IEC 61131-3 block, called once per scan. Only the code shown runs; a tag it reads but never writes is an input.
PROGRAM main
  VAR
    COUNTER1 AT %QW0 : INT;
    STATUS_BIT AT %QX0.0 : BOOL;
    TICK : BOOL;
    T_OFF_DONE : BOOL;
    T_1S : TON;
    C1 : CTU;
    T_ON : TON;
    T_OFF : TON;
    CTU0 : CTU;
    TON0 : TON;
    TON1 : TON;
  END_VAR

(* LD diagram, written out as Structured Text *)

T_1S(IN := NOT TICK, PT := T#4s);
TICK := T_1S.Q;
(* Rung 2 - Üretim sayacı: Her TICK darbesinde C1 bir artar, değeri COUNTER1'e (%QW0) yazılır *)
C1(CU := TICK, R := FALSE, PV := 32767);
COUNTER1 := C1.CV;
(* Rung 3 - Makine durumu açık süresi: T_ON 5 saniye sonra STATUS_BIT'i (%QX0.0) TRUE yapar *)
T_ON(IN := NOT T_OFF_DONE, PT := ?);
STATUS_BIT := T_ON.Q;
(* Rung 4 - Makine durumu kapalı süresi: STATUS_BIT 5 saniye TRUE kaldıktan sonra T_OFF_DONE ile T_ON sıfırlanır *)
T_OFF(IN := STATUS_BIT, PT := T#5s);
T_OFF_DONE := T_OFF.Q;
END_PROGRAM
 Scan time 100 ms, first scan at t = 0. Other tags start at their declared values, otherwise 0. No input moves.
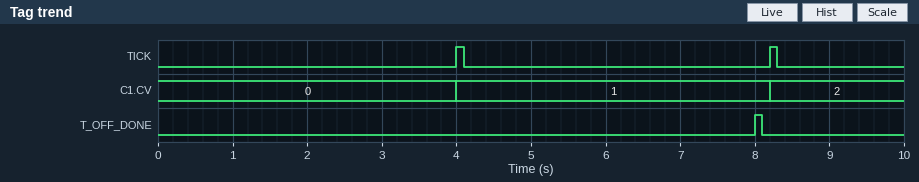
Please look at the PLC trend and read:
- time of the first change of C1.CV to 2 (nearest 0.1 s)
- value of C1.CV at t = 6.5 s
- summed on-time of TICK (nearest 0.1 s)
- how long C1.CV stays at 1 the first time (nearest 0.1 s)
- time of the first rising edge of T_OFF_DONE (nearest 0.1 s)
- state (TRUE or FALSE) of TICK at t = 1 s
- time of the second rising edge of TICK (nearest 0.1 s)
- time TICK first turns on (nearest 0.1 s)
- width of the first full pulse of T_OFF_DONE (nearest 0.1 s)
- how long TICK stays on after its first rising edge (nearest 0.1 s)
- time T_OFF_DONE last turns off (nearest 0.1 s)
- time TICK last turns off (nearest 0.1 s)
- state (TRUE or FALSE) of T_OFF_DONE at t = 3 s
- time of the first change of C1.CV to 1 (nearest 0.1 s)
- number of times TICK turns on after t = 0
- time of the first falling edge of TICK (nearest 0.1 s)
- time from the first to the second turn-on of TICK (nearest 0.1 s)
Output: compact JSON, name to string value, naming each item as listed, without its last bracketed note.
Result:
{"time of the first change of C1.CV to 2": "8.2 s", "value of C1.CV at t = 6.5 s": "1", "summed on-time of TICK": "0.2 s", "how long C1.CV stays at 1 the first time": "4.2 s", "time of the first rising edge of T_OFF_DONE": "8.0 s", "state (TRUE or FALSE) of TICK at t = 1 s": "FALSE", "time of the second rising edge of TICK": "8.2 s", "time TICK first turns on": "4.0 s", "width of the first full pulse of T_OFF_DONE": "0.1 s", "how long TICK stays on after its first rising edge": "0.1 s", "time T_OFF_DONE last turns off": "8.1 s", "time TICK last turns off": "8.3 s", "state (TRUE or FALSE) of T_OFF_DONE at t = 3 s": "FALSE", "time of the first change of C1.CV to 1": "4.0 s", "number of times TICK turns on after t = 0": "2", "time of the first falling edge of TICK": "4.1 s", "time from the first to the second turn-on of TICK": "4.2 s"}
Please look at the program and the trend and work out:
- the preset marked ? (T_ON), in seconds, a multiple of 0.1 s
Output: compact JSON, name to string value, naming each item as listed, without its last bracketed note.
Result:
{"the preset marked ? (T_ON), in seconds, a multiple of 0.1 s": "3.0 s"}
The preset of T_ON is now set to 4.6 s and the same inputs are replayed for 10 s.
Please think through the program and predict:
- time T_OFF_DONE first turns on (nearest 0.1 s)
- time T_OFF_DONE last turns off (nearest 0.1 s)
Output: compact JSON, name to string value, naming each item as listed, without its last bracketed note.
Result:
{"time T_OFF_DONE first turns on": "9.6 s", "time T_OFF_DONE last turns off": "9.7 s"}
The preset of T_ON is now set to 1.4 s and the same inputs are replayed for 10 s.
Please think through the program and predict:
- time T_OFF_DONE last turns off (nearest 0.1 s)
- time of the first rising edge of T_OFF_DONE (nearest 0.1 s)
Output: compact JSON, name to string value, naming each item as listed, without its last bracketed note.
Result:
{"time T_OFF_DONE last turns off": "6.5 s", "time of the first rising edge of T_OFF_DONE": "6.4 s"}
